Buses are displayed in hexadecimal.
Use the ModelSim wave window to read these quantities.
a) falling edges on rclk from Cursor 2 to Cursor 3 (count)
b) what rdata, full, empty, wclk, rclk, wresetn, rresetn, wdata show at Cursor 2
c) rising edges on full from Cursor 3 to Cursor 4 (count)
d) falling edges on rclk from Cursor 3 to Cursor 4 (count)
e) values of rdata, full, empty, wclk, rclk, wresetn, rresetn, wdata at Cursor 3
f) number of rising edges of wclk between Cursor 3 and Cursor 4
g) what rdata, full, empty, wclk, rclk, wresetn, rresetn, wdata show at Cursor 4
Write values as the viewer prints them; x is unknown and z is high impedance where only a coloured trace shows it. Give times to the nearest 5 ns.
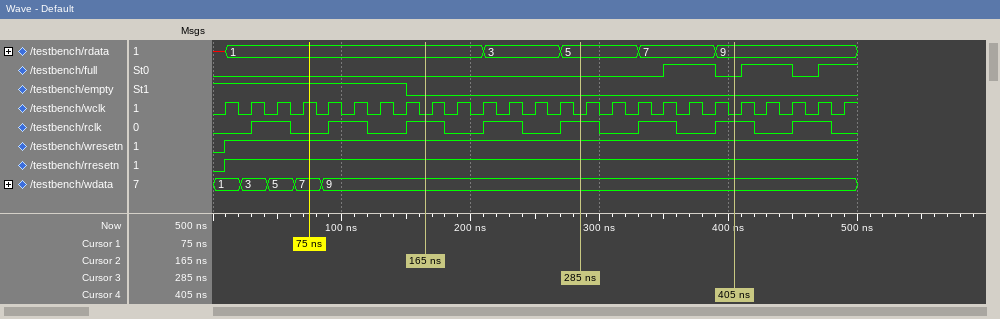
2
rdata=1, full=0, empty=0, wclk=0, rclk=1, wresetn=1, rresetn=1, wdata=9
1
2
rdata=5, full=0, empty=0, wclk=0, rclk=1, wresetn=1, rresetn=1, wdata=9
6
rdata=9, full=0, empty=0, wclk=0, rclk=1, wresetn=1, rresetn=1, wdata=9
